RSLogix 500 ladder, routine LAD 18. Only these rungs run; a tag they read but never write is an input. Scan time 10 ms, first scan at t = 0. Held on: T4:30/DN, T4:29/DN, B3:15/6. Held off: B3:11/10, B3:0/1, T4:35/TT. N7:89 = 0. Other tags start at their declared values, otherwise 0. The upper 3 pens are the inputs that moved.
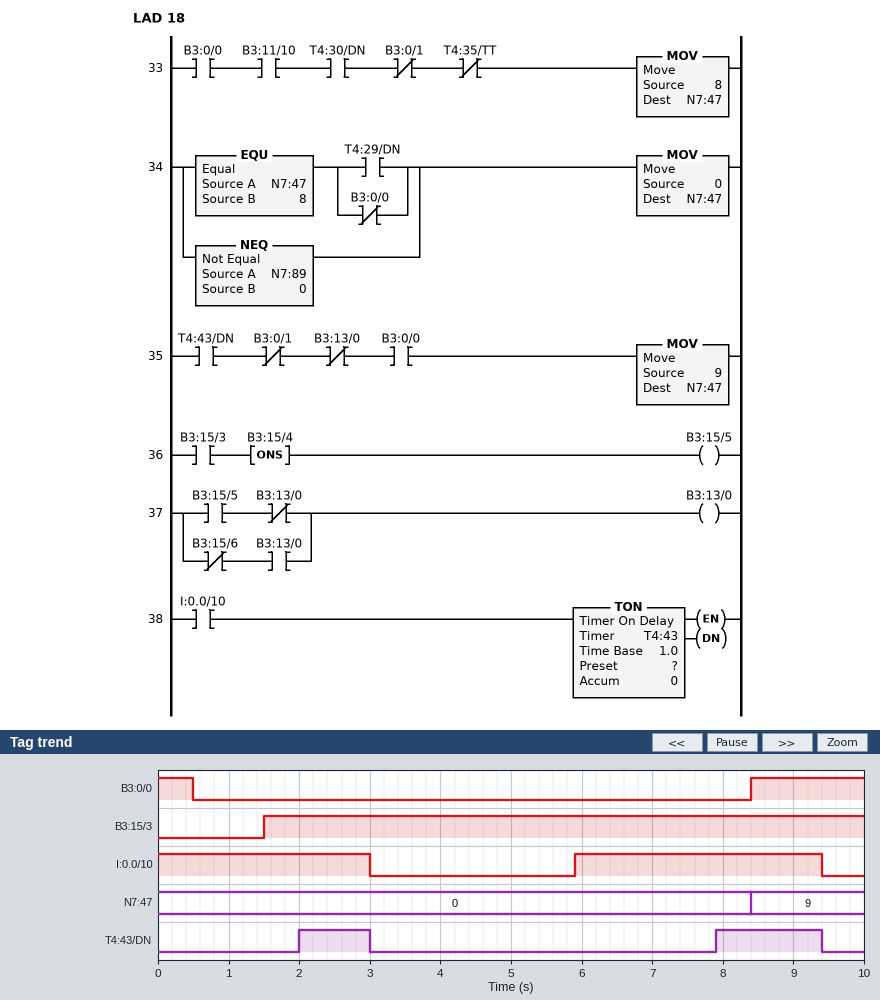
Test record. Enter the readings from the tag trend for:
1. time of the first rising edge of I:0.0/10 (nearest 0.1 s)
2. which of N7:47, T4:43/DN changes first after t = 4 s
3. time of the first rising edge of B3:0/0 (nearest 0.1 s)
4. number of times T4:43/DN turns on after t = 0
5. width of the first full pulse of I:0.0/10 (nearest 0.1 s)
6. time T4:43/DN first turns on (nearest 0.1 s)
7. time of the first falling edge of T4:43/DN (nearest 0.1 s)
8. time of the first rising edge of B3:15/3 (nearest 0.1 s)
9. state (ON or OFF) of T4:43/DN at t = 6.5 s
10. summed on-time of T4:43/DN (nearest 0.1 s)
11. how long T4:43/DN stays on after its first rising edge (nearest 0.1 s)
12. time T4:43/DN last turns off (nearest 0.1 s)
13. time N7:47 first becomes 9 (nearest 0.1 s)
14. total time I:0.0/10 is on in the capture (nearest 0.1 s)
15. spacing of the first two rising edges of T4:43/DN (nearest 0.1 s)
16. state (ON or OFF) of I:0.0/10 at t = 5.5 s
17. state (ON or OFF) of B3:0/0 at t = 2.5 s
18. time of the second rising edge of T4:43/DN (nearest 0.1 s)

5.9 s
T4:43/DN
8.4 s
2
3.5 s
2.0 s
3.0 s
1.5 s
OFF
2.5 s
1.0 s
9.4 s
8.4 s
6.5 s
5.9 s
OFF
OFF
7.9 s
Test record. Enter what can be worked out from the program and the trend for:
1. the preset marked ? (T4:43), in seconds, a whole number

2 s
